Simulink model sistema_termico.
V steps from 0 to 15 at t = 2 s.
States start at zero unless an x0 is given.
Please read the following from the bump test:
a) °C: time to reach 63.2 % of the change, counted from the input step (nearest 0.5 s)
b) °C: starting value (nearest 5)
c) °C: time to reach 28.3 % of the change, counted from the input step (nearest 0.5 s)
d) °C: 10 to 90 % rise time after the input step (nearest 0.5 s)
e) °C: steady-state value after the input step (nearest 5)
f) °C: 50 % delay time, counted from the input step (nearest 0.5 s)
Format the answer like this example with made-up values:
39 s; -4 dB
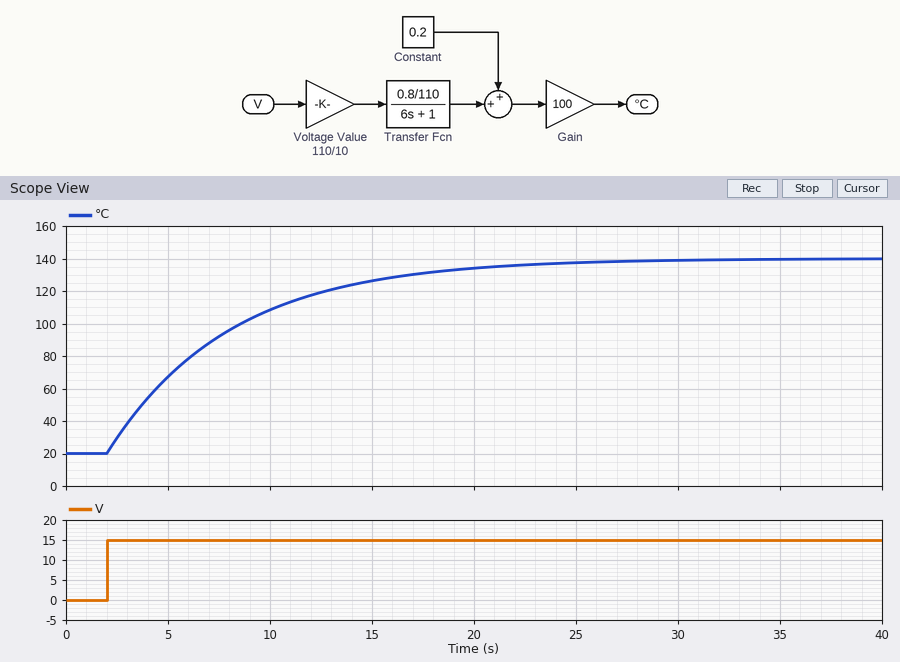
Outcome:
6.0 s; 20; 2.0 s; 13.0 s; 140; 4.0 s
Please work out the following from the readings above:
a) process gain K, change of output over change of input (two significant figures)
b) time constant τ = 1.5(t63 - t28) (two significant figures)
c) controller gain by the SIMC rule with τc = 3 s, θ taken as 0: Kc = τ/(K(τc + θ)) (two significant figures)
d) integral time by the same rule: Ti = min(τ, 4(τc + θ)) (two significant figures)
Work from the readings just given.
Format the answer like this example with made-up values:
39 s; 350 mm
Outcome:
8.0; 6.0 s; 0.25; 6.0 s
